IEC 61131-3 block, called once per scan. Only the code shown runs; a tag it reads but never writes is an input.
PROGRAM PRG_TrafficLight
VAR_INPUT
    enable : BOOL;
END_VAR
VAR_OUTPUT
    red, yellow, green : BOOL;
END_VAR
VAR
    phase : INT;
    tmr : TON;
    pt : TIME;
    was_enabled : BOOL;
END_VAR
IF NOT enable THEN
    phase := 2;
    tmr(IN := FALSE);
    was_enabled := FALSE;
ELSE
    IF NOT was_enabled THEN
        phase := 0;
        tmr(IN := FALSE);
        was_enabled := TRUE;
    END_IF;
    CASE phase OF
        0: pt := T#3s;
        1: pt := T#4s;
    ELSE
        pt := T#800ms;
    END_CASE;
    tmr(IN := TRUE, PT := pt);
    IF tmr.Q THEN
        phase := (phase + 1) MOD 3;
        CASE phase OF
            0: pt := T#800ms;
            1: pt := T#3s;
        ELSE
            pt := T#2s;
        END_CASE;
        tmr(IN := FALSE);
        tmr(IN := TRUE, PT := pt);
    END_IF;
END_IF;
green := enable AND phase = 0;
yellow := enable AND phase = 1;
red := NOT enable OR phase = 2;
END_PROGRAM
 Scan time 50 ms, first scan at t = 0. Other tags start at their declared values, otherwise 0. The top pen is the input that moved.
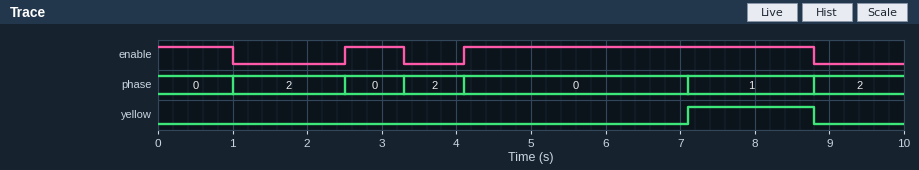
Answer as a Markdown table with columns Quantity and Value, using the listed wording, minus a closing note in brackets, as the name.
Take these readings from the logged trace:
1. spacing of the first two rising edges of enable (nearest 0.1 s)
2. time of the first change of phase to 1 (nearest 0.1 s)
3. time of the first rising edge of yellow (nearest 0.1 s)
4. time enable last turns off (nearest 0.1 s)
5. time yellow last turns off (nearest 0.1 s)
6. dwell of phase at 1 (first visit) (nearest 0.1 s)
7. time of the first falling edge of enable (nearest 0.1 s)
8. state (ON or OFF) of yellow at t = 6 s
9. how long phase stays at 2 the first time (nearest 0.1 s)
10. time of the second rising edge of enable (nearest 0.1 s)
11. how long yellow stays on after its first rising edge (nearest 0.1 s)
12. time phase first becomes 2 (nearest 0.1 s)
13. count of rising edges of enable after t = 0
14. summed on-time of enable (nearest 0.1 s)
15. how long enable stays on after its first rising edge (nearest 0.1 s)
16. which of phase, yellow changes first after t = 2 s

| Quantity | Value |
|---|---|
| spacing of the first two rising edges of enable | 1.6 s |
| time of the first change of phase to 1 | 7.1 s |
| time of the first rising edge of yellow | 7.1 s |
| time enable last turns off | 8.8 s |
| time yellow last turns off | 8.8 s |
| dwell of phase at 1 (first visit) | 1.7 s |
| time of the first falling edge of enable | 1.0 s |
| state (ON or OFF) of yellow at t = 6 s | OFF |
| how long phase stays at 2 the first time | 1.5 s |
| time of the second rising edge of enable | 4.1 s |
| how long yellow stays on after its first rising edge | 1.7 s |
| time phase first becomes 2 | 1.0 s |
| count of rising edges of enable after t = 0 | 2 |
| summed on-time of enable | 6.5 s |
| how long enable stays on after its first rising edge | 0.8 s |
| which of phase, yellow changes first after t = 2 s | phase |
